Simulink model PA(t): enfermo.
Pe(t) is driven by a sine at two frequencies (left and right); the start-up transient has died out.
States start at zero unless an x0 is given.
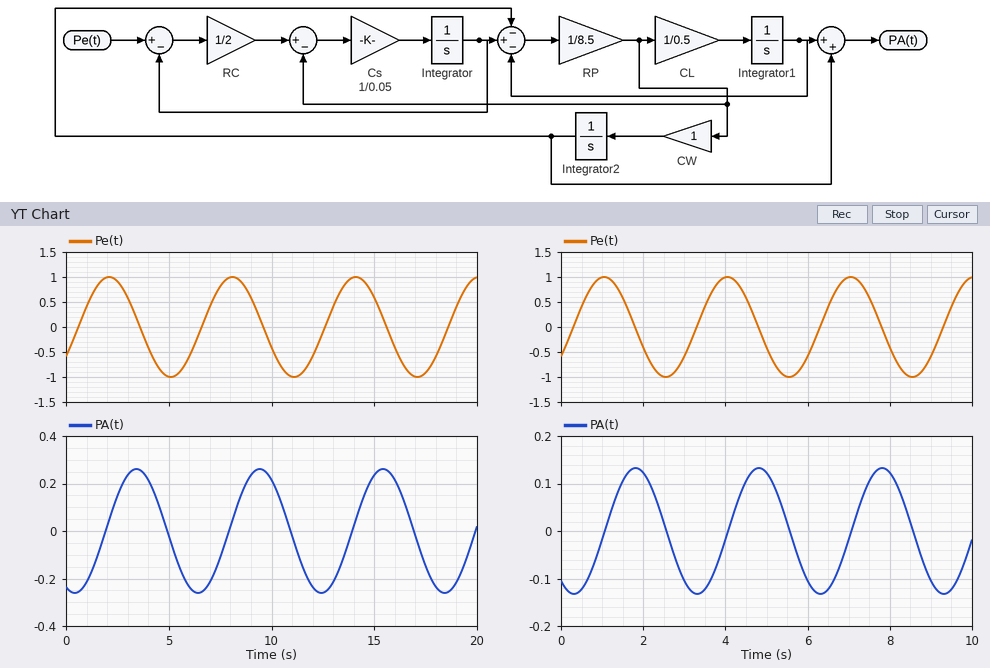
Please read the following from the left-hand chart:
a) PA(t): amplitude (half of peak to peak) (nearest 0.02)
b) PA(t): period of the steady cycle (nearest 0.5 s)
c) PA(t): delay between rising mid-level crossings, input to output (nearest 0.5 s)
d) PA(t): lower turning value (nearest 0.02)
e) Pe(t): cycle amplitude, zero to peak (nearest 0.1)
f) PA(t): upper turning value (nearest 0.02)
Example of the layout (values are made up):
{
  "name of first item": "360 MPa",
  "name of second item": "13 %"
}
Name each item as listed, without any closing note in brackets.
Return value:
{
  "PA(t): amplitude (half of peak to peak)": "0.26",
  "PA(t): period of the steady cycle": "6.0 s",
  "PA(t): delay between rising mid-level crossings, input to output": "1.5 s",
  "PA(t): lower turning value": "-0.26",
  "Pe(t): cycle amplitude, zero to peak": "1.0",
  "PA(t): upper turning value": "0.26"
}
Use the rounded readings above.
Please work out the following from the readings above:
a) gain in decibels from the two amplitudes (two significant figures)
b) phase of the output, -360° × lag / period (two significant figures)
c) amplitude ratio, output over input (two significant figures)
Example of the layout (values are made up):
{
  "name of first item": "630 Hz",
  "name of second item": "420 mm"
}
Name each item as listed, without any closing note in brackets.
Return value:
{
  "gain in decibels from the two amplitudes": "-12 dB",
  "phase of the output, -360° × lag / period": "-90°",
  "amplitude ratio, output over input": "0.26"
}
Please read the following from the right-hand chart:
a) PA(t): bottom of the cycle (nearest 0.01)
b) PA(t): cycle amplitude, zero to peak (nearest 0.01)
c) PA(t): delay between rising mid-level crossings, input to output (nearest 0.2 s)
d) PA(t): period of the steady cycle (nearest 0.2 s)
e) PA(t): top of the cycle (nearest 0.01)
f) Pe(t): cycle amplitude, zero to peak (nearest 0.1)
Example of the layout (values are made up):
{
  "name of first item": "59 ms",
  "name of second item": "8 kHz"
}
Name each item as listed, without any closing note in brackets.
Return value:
{
  "PA(t): bottom of the cycle": "-0.13",
  "PA(t): cycle amplitude, zero to peak": "0.13",
  "PA(t): delay between rising mid-level crossings, input to output": "0.8 s",
  "PA(t): period of the steady cycle": "3.0 s",
  "PA(t): top of the cycle": "0.13",
  "Pe(t): cycle amplitude, zero to peak": "1.0"
}
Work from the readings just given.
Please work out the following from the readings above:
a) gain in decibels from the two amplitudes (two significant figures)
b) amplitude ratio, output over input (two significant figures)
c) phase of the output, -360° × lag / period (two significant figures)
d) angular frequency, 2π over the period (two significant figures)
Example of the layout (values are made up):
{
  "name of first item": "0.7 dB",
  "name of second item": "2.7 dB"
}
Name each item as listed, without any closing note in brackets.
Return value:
{
  "gain in decibels from the two amplitudes": "-18 dB",
  "amplitude ratio, output over input": "0.13",
  "phase of the output, -360° × lag / period": "-96°",
  "angular frequency, 2π over the period": "2.1 rad/s"
}
